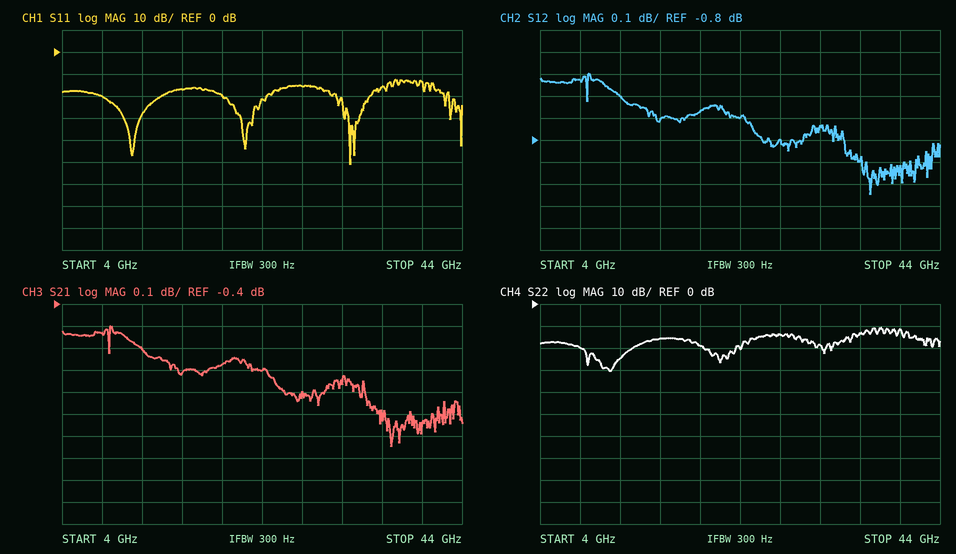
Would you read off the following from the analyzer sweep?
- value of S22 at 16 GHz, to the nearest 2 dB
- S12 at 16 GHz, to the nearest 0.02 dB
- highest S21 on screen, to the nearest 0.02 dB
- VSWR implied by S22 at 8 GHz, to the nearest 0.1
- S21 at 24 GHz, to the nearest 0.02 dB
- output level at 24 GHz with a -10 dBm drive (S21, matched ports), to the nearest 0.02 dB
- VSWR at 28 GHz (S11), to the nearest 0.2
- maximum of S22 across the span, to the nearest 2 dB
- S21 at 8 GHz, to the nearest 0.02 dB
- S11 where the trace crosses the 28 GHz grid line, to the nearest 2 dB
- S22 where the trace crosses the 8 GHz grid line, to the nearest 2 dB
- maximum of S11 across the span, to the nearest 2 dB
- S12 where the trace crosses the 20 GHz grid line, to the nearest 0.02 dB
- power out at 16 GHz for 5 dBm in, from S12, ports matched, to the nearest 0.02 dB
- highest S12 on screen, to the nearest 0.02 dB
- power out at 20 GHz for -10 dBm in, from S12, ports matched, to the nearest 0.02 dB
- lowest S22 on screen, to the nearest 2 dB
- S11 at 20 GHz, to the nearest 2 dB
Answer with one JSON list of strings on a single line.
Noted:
["-16 dB", "-0.70 dB", "-0.50 dB", "1.2", "-0.70 dB", "-10.70 dBm", "1.4", "-10 dB", "-0.54 dB", "-16 dB", "-20 dB", "-12 dB", "-0.68 dB", "4.30 dBm", "-0.50 dB", "-10.68 dBm", "-30 dB", "-20 dB"]
